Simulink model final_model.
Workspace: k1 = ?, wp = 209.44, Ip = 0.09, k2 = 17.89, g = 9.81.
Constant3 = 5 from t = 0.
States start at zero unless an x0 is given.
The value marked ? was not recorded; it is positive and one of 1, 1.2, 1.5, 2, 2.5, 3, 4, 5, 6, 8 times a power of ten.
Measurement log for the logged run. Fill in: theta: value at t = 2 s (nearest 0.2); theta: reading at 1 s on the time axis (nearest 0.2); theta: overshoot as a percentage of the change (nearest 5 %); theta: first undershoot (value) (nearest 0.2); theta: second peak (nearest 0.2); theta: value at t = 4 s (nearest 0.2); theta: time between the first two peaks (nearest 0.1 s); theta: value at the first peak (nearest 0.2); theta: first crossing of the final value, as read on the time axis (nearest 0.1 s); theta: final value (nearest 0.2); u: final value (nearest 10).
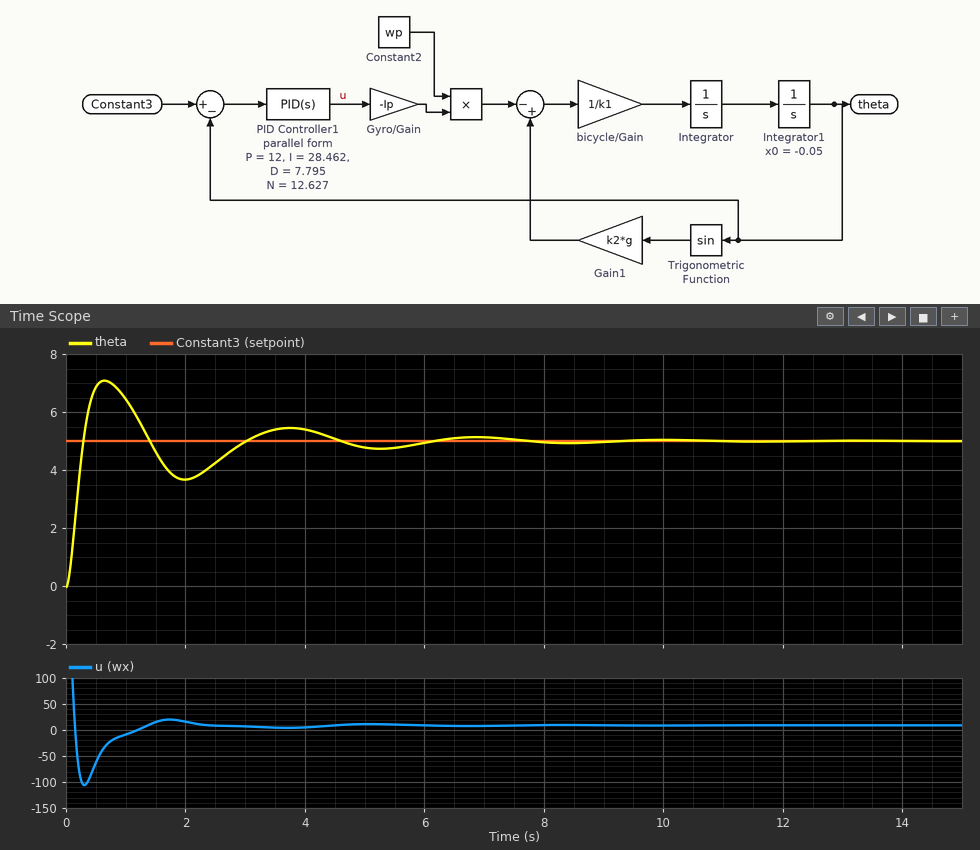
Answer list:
3.6
6.4
40 %
3.6
5.4
5.4
3.1 s
7.0
0.3 s
5.0
10
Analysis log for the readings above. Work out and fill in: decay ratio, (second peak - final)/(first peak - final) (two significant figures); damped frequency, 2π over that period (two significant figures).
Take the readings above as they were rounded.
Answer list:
0.20
2.0 rad/s
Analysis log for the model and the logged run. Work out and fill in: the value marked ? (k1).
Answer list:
30
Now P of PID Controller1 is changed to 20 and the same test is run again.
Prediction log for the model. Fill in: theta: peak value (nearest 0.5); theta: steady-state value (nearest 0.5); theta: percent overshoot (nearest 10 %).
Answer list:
7.5
5.0
50 %
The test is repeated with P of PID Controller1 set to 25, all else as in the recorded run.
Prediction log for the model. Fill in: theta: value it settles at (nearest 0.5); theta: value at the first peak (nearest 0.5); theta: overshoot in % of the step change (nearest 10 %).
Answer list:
5.0
7.5
50 %
